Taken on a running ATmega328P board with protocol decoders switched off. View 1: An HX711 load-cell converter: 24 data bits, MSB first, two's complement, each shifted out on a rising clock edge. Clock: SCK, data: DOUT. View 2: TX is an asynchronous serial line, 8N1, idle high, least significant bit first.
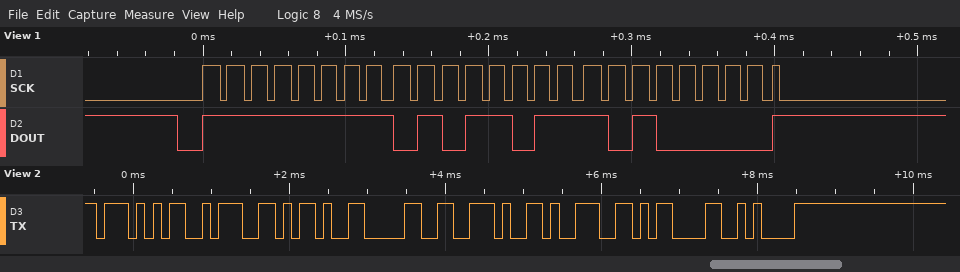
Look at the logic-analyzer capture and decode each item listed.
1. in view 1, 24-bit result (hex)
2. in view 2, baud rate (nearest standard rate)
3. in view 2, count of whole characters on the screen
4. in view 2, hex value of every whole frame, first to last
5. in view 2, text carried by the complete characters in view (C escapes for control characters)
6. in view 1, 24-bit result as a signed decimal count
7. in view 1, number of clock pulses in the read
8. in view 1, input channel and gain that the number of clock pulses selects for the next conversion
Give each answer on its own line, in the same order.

0xFF5BA0
9600 baud
8
57 3A 2D 30 2E 39 0D 0A
"W:-0.9\r\n"
-42080
25
channel A, gain 128
